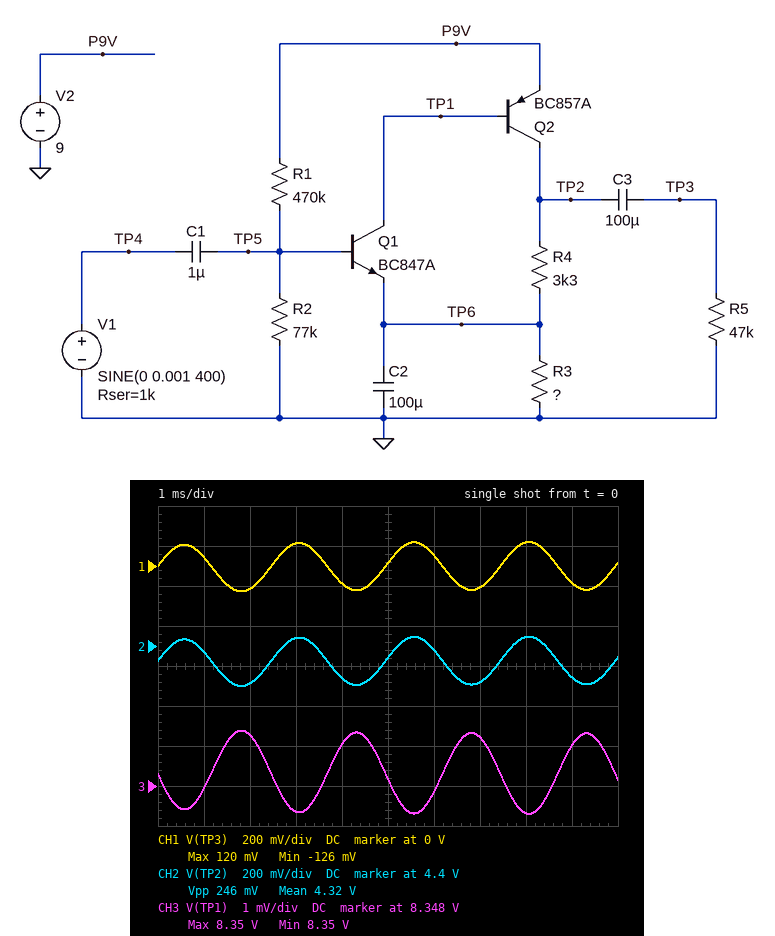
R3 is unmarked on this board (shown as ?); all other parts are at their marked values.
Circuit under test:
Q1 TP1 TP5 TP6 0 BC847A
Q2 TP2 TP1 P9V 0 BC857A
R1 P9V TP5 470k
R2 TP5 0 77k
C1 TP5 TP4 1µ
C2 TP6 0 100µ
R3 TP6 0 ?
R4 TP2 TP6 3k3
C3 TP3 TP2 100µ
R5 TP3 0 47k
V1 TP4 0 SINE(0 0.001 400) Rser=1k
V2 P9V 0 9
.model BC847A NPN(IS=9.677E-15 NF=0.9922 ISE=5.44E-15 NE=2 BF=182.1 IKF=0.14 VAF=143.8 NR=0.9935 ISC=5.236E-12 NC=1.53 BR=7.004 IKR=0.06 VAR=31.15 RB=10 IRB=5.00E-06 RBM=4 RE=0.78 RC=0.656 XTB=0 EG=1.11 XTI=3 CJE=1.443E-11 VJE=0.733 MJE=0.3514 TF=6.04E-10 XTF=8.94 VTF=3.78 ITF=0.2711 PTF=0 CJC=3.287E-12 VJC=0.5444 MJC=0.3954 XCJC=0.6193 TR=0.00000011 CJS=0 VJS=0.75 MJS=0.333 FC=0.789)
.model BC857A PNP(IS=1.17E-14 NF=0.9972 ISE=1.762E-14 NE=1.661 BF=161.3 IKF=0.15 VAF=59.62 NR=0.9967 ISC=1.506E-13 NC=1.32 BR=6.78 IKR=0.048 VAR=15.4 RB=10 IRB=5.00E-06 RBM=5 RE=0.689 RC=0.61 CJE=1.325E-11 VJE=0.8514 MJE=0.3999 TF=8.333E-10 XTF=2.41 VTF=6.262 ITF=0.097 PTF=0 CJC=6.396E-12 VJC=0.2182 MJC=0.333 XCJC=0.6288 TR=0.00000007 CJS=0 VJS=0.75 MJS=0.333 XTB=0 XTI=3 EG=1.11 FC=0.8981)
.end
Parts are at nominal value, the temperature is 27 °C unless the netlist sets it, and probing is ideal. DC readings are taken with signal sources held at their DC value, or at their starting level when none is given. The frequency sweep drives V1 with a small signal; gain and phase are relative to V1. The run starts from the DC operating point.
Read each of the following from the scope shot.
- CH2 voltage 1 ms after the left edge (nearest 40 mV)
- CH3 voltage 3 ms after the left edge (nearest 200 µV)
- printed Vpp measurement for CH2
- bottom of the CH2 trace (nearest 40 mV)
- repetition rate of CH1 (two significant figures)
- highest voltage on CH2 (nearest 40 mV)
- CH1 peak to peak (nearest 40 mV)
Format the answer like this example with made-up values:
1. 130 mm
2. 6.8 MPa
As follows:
1. 4.36 V
2. 8.3474 V
3. 246 mV
4. 4.20 V
5. 400 Hz
6. 4.44 V
7. 240 mV
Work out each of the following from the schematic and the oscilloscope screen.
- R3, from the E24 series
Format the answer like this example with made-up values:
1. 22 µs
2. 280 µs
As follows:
1. 680 Ω
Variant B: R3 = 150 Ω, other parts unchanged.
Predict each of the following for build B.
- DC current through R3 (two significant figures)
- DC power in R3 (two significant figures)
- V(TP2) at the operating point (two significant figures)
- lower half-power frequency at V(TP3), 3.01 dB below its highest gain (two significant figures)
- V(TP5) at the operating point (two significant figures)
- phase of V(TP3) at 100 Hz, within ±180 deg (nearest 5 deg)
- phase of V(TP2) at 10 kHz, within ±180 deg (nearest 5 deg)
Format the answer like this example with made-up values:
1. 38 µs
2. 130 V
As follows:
1. 3.1 mA
2. 1.4 mW
3. 9.0 V
4. 48 Hz
5. 1.1 V
6. 25 deg
7. 0 deg
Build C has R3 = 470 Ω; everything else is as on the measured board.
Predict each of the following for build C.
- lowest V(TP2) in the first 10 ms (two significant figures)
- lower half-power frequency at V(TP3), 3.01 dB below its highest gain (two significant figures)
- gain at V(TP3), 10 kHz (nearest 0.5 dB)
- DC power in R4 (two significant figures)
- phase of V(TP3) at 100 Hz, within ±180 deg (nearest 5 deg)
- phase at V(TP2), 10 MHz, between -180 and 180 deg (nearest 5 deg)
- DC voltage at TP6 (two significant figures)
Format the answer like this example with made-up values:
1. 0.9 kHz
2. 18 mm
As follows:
1. 5.7 V
2. 86 Hz
3. 44.5 dB
4. 7.9 mW
5. 40 deg
6. -160 deg
7. 730 mV
